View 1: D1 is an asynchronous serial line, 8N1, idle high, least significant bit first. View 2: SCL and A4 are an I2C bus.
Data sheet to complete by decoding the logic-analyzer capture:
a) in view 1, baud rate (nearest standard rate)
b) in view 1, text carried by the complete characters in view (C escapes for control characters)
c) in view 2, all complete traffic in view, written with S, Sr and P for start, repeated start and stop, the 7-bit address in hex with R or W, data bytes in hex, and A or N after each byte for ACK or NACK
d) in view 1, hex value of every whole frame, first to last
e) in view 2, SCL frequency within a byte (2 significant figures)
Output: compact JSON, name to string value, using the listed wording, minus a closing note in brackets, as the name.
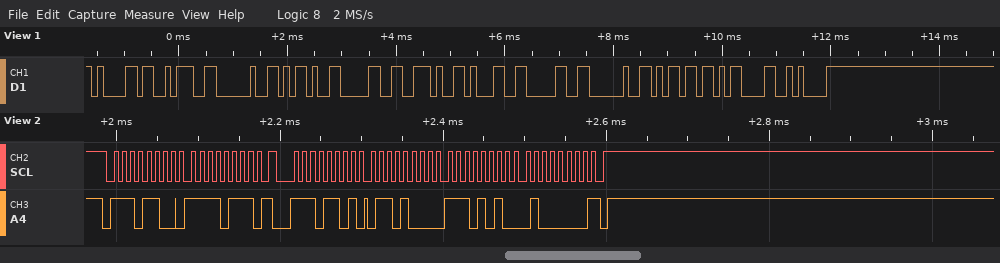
{"in view 1, baud rate": "9600 baud", "in view 1, text carried by the complete characters in view": "\"a: -0.10 m\\r\\n\"", "in view 2, all complete traffic in view, written with S, Sr and P for start, repeated start and stop, the 7-bit address in hex with R or W, data bytes in hex, and A or N after each byte for ACK or NACK": "S 76W A F7 A Sr 76R A 68 A EA A 40 N P", "in view 1, hex value of every whole frame, first to last": "61 3A 20 2D 30 2E 31 30 20 6D 0D 0A", "in view 2, SCL frequency within a byte": "100 kHz"}
